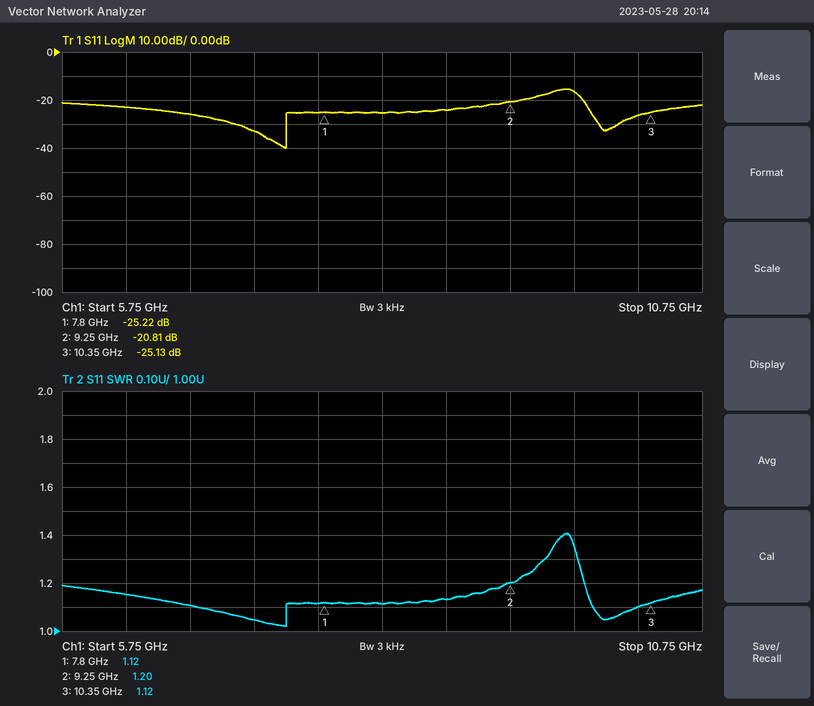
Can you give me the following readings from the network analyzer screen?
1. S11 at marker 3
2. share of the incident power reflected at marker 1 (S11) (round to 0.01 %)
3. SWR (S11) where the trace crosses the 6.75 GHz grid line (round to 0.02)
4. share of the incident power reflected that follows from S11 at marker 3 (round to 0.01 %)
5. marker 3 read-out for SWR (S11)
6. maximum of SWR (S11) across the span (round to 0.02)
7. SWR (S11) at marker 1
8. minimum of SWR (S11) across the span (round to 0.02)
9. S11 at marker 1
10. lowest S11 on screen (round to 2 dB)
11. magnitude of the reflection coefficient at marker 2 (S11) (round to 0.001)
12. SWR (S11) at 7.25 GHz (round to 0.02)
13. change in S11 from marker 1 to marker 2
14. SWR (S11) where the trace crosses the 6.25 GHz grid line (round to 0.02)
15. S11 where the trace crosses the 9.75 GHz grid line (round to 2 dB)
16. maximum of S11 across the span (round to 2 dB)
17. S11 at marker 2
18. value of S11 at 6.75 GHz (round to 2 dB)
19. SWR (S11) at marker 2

-25.13 dB
0.30 %
1.10
0.31 %
1.12
1.40
1.12
1.02
-25.22 dB
-40 dB
0.091
1.04
4.41 dB
1.16
-16 dB
-16 dB
-20.81 dB
-26 dB
1.20
